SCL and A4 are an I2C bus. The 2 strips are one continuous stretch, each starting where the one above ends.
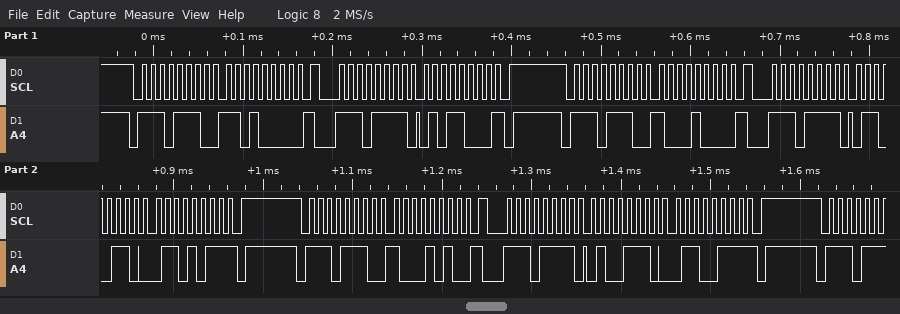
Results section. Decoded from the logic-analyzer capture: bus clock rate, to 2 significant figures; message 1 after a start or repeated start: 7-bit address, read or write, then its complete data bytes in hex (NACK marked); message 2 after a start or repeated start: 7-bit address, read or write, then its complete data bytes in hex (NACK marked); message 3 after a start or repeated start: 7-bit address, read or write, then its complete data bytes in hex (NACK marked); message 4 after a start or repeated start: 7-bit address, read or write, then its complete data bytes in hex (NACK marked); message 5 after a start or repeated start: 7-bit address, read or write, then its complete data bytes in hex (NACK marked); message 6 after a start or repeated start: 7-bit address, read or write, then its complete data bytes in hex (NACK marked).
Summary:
100 kHz
0x77 write: D0
0x77 read: 58 NACK
0x77 write: 88
0x77 read: 66 6B NACK
0x77 write: 8A
0x77 read: 4E 67 NACK
